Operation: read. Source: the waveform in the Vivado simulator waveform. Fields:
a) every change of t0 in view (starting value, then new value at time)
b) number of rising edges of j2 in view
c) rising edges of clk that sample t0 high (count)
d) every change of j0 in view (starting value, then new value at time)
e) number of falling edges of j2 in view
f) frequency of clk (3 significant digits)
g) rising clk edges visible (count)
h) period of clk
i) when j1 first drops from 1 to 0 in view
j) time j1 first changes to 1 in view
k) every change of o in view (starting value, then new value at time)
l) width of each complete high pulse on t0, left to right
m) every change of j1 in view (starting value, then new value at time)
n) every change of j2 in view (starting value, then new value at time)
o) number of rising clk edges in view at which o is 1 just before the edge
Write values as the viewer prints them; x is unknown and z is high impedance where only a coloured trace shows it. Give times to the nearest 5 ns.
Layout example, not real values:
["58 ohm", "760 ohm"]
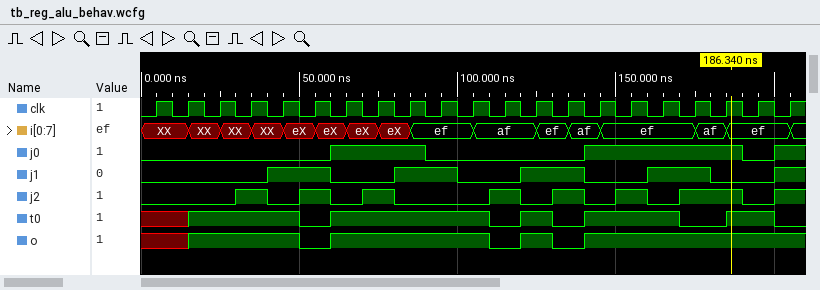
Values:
["x, 1 at 15 ns, 0 at 50 ns, 1 at 60 ns, 0 at 110 ns, 1 at 120 ns, 0 at 130 ns, 1 at 140 ns, 0 at 170 ns, 1 at 185 ns, 0 at 200 ns", "8", "13", "0, 1 at 60 ns, 0 at 90 ns, 1 at 140 ns, 0 at 190 ns, 1 at 200 ns", "7", "100 MHz", "21", "10 ns", "60 ns", "40 ns", "x, 1 at 15 ns, 0 at 50 ns, 1 at 60 ns, 0 at 110 ns, 1 at 120 ns, 0 at 130 ns, 1 at 140 ns", "50 ns, 10 ns, 30 ns, 15 ns", "0, 1 at 40 ns, 0 at 60 ns, 1 at 80 ns, 0 at 100 ns, 1 at 120 ns, 0 at 140 ns, 1 at 160 ns, 0 at 180 ns, 1 at 200 ns", "0, 1 at 30 ns, 0 at 40 ns, 1 at 50 ns, 0 at 60 ns, 1 at 70 ns, 0 at 80 ns, 1 at 110 ns, 0 at 120 ns, 1 at 130 ns, 0 at 140 ns, 1 at 150 ns, 0 at 160 ns, 1 at 170 ns, 0 at 190 ns, 1 at 200 ns", "16"]
